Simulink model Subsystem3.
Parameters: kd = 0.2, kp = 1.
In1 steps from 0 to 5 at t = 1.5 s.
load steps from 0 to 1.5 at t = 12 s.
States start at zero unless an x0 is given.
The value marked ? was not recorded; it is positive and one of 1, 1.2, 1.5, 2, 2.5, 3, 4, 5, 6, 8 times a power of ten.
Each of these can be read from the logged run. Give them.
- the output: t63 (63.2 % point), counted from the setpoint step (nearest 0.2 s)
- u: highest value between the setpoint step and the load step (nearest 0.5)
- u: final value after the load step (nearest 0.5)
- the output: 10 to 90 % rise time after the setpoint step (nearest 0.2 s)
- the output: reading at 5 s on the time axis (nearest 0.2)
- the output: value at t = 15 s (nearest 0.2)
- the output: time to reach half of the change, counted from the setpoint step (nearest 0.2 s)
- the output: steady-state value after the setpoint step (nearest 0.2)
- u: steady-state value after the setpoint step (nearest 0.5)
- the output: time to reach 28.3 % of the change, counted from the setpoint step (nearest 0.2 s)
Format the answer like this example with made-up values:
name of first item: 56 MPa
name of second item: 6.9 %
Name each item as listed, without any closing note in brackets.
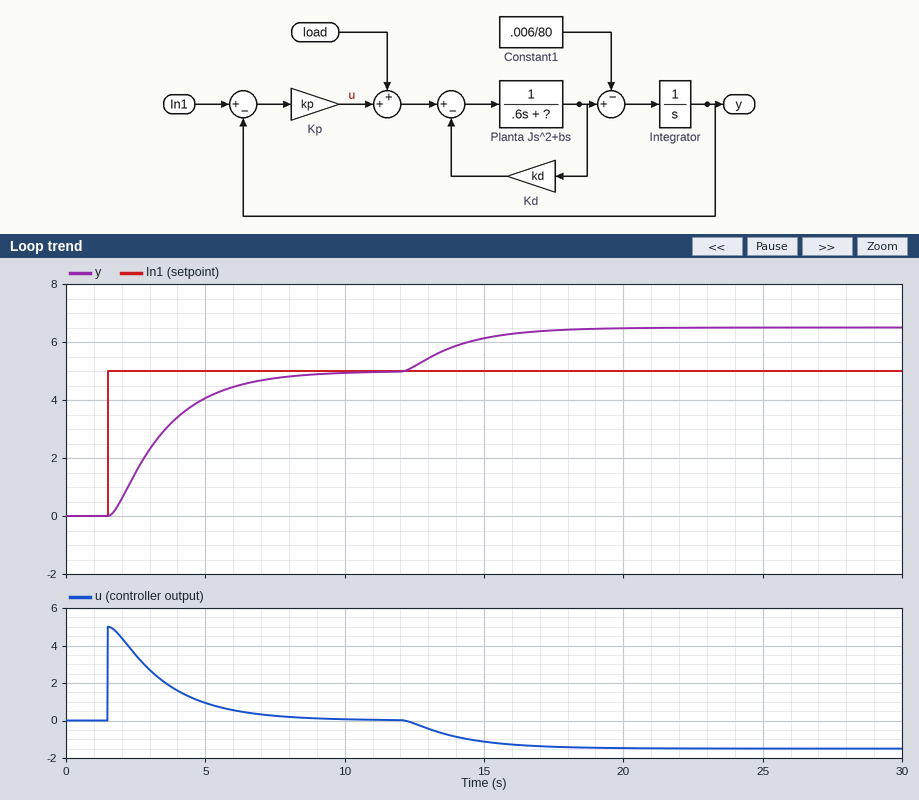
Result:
the output: t63 (63.2 % point), counted from the setpoint step: 2.2 s
u: highest value between the setpoint step and the load step: 5.0
u: final value after the load step: -1.5
the output: 10 to 90 % rise time after the setpoint step: 4.2 s
the output: reading at 5 s on the time axis: 4.0
the output: value at t = 15 s: 6.2
the output: time to reach half of the change, counted from the setpoint step: 1.6 s
the output: steady-state value after the setpoint step: 5.0
u: steady-state value after the setpoint step: 0.0
the output: time to reach 28.3 % of the change, counted from the setpoint step: 1.0 s
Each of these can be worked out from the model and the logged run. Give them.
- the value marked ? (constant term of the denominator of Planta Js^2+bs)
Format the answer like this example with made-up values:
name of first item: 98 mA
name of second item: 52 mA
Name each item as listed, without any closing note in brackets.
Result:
the value marked ?: 2
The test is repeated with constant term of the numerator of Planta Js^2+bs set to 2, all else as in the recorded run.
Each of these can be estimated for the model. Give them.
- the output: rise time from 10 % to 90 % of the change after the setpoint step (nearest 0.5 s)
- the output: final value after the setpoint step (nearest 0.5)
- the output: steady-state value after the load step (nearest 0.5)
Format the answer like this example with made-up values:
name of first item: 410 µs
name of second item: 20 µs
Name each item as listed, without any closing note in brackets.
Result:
the output: rise time from 10 % to 90 % of the change after the setpoint step: 2.0 s
the output: final value after the setpoint step: 5.0
the output: steady-state value after the load step: 6.5
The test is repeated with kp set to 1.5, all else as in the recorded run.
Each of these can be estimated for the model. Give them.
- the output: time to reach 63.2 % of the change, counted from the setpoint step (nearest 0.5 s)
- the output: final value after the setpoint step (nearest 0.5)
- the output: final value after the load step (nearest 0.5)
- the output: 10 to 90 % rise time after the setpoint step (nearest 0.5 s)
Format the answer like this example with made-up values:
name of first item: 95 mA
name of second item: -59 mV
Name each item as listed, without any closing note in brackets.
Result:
the output: time to reach 63.2 % of the change, counted from the setpoint step: 1.5 s
the output: final value after the setpoint step: 5.0
the output: final value after the load step: 6.0
the output: 10 to 90 % rise time after the setpoint step: 2.5 s
